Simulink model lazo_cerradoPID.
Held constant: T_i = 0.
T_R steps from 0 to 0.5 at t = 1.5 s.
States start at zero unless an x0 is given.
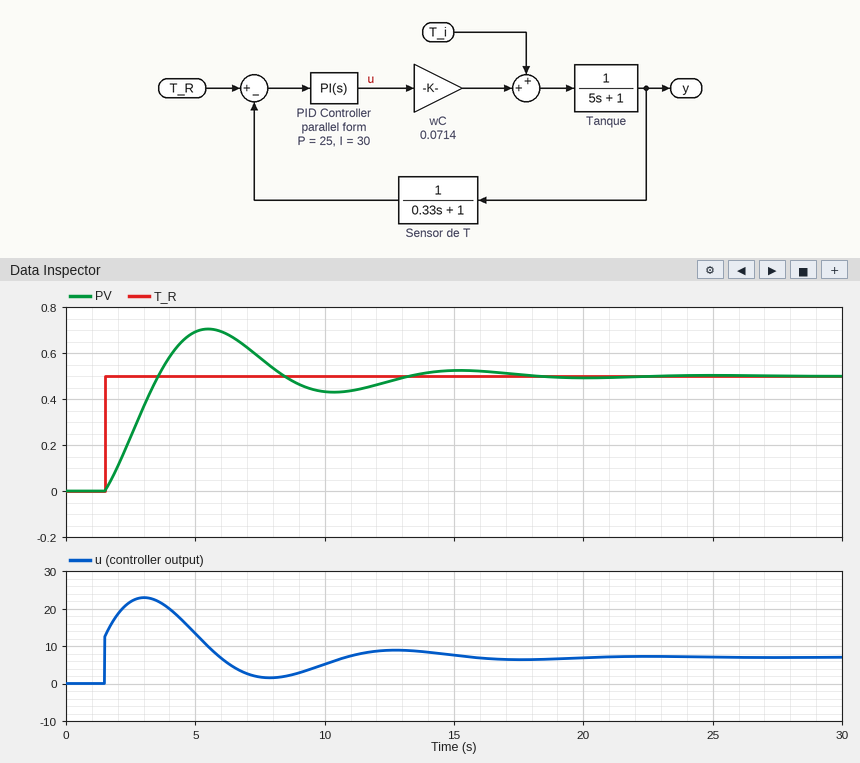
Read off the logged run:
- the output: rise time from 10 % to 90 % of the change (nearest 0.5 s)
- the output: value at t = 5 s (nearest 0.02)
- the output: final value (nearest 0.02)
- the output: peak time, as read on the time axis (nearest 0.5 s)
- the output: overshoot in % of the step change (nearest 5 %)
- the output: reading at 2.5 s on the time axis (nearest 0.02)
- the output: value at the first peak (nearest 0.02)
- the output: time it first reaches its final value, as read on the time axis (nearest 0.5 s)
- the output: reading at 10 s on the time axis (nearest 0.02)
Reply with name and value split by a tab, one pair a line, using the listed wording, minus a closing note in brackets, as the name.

the output: rise time from 10 % to 90 % of the change	1.5 s
the output: value at t = 5 s	0.70
the output: final value	0.50
the output: peak time, as read on the time axis	5.5 s
the output: overshoot in % of the step change	40 %
the output: reading at 2.5 s on the time axis	0.24
the output: value at the first peak	0.70
the output: time it first reaches its final value, as read on the time axis	3.5 s
the output: reading at 10 s on the time axis	0.44
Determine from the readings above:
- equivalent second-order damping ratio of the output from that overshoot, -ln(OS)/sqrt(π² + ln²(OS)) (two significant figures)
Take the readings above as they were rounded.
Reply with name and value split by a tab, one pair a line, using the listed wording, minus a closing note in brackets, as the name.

equivalent second-order damping ratio of the output from that overshoot, -ln(OS)/sqrt(π² + ln²(OS))	0.28
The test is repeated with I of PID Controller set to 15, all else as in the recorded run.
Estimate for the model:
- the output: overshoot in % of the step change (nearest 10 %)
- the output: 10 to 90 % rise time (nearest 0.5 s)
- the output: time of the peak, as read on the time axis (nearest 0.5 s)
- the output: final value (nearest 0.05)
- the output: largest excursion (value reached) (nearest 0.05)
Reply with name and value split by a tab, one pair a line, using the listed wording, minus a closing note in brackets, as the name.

the output: overshoot in % of the step change	20 %
the output: 10 to 90 % rise time	2.5 s
the output: time of the peak, as read on the time axis	7.0 s
the output: final value	0.50
the output: largest excursion (value reached)	0.60
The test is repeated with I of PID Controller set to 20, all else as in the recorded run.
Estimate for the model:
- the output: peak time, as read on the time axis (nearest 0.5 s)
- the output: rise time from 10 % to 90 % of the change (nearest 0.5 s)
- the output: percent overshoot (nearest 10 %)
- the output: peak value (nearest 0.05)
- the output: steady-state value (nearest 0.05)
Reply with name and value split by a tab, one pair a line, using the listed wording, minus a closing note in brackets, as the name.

the output: peak time, as read on the time axis	6.5 s
the output: rise time from 10 % to 90 % of the change	2.0 s
the output: percent overshoot	30 %
the output: peak value	0.65
the output: steady-state value	0.50
